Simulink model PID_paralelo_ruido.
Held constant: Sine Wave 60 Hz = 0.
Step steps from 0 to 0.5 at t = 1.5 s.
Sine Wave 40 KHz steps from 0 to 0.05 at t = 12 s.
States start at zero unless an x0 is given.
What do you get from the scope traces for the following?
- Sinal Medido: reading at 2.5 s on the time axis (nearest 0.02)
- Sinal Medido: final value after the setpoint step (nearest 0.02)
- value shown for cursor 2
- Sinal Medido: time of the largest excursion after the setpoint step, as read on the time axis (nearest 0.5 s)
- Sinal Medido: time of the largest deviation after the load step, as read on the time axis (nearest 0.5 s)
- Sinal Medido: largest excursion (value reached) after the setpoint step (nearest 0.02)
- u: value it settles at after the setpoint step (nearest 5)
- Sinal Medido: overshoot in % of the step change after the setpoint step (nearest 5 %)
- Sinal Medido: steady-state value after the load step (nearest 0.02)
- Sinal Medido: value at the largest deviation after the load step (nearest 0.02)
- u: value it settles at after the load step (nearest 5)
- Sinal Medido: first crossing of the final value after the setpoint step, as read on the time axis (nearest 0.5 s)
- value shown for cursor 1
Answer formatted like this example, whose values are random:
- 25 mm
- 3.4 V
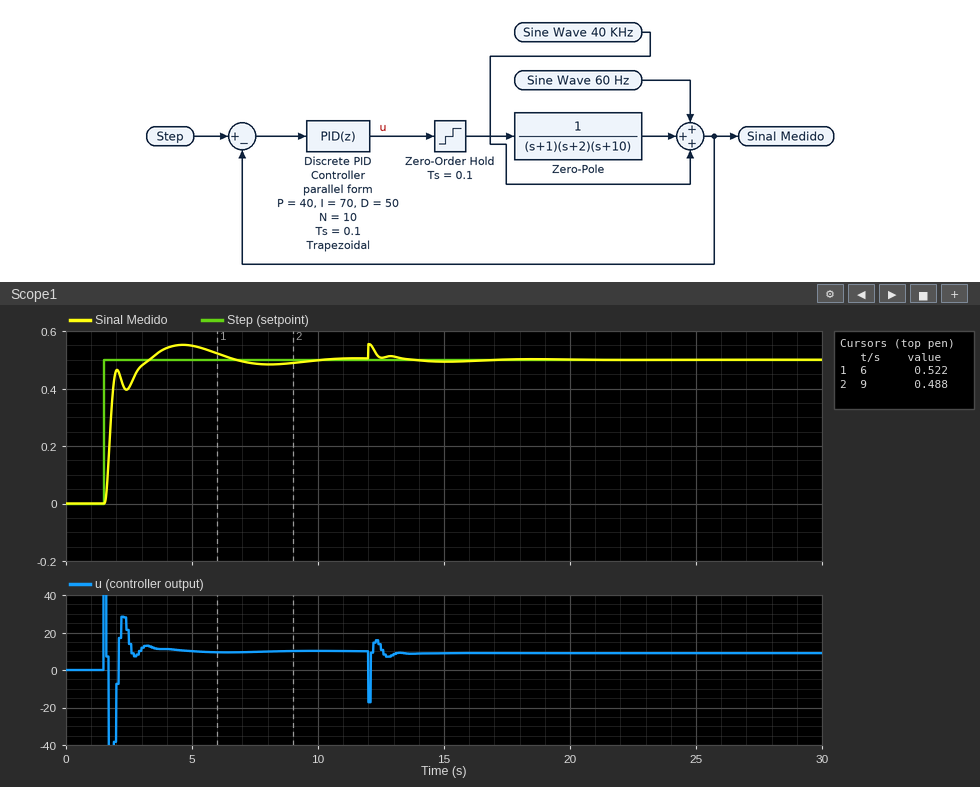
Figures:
- 0.40
- 0.50
- 0.488
- 4.5 s
- 12.0 s
- 0.56
- 10
- 10 %
- 0.50
- 0.56
- 10
- 3.5 s
- 0.522
